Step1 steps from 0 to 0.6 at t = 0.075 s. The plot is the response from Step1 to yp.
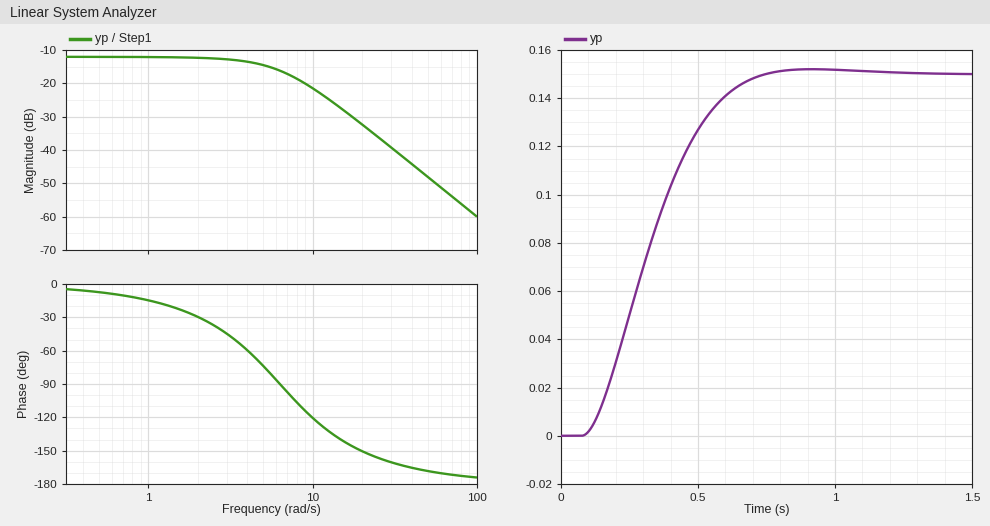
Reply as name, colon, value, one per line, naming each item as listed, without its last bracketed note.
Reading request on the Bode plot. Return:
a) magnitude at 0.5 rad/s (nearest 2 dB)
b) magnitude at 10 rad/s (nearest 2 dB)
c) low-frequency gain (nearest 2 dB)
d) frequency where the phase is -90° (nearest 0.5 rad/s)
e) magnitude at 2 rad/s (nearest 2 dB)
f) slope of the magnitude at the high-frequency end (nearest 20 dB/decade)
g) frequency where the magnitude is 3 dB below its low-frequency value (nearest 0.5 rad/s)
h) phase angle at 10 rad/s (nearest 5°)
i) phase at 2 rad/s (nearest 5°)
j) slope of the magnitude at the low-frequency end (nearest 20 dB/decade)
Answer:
magnitude at 0.5 rad/s: -12 dB
magnitude at 10 rad/s: -22 dB
low-frequency gain: -12 dB
frequency where the phase is -90°: 6.5 rad/s
magnitude at 2 rad/s: -12 dB
slope of the magnitude at the high-frequency end: -40 dB/decade
frequency where the magnitude is 3 dB below its low-frequency value: 5.5 rad/s
phase angle at 10 rad/s: -120°
phase at 2 rad/s: -30°
slope of the magnitude at the low-frequency end: 0 dB/decade
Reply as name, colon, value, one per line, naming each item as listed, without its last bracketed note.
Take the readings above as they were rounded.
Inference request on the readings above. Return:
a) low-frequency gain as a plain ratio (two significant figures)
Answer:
low-frequency gain as a plain ratio: 0.25
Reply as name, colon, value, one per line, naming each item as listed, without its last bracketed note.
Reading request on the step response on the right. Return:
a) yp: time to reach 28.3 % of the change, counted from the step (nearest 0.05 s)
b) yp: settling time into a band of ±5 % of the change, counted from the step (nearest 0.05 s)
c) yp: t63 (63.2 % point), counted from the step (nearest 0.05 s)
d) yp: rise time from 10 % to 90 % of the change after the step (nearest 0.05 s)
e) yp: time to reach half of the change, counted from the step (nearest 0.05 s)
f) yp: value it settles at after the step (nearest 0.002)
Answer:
yp: time to reach 28.3 % of the change, counted from the step: 0.15 s
yp: settling time into a band of ±5 % of the change, counted from the step: 0.55 s
yp: t63 (63.2 % point), counted from the step: 0.30 s
yp: rise time from 10 % to 90 % of the change after the step: 0.40 s
yp: time to reach half of the change, counted from the step: 0.25 s
yp: value it settles at after the step: 0.150
